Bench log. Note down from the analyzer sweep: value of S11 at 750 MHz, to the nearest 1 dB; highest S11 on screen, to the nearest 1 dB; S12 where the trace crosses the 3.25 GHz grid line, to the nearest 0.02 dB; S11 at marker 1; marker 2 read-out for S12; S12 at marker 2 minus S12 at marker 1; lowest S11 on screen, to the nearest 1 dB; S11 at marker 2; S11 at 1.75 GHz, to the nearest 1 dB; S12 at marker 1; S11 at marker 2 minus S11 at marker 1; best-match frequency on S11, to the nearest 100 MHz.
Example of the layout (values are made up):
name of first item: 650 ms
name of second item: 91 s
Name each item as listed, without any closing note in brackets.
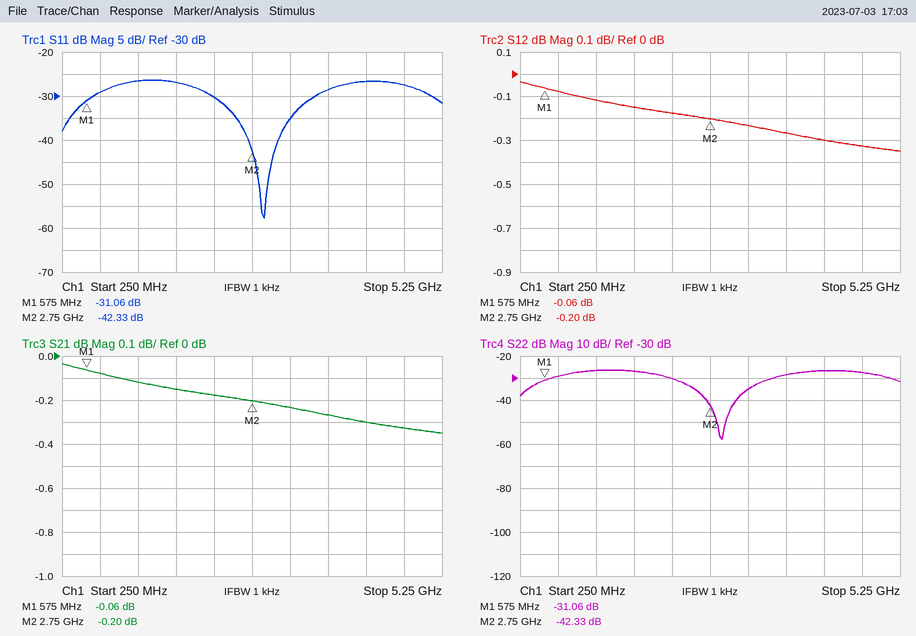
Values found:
value of S11 at 750 MHz, to the nearest 1 dB: -29 dB
highest S11 on screen, to the nearest 1 dB: -26 dB
S12 where the trace crosses the 3.25 GHz grid line, to the nearest 0.02 dB: -0.24 dB
S11 at marker 1: -31.06 dB
marker 2 read-out for S12: -0.20 dB
S12 at marker 2 minus S12 at marker 1: -0.14 dB
lowest S11 on screen, to the nearest 1 dB: -58 dB
S11 at marker 2: -42.33 dB
S11 at 1.75 GHz, to the nearest 1 dB: -27 dB
S12 at marker 1: -0.06 dB
S11 at marker 2 minus S11 at marker 1: -11.27 dB
best-match frequency on S11, to the nearest 100 MHz: 2.9 GHz
